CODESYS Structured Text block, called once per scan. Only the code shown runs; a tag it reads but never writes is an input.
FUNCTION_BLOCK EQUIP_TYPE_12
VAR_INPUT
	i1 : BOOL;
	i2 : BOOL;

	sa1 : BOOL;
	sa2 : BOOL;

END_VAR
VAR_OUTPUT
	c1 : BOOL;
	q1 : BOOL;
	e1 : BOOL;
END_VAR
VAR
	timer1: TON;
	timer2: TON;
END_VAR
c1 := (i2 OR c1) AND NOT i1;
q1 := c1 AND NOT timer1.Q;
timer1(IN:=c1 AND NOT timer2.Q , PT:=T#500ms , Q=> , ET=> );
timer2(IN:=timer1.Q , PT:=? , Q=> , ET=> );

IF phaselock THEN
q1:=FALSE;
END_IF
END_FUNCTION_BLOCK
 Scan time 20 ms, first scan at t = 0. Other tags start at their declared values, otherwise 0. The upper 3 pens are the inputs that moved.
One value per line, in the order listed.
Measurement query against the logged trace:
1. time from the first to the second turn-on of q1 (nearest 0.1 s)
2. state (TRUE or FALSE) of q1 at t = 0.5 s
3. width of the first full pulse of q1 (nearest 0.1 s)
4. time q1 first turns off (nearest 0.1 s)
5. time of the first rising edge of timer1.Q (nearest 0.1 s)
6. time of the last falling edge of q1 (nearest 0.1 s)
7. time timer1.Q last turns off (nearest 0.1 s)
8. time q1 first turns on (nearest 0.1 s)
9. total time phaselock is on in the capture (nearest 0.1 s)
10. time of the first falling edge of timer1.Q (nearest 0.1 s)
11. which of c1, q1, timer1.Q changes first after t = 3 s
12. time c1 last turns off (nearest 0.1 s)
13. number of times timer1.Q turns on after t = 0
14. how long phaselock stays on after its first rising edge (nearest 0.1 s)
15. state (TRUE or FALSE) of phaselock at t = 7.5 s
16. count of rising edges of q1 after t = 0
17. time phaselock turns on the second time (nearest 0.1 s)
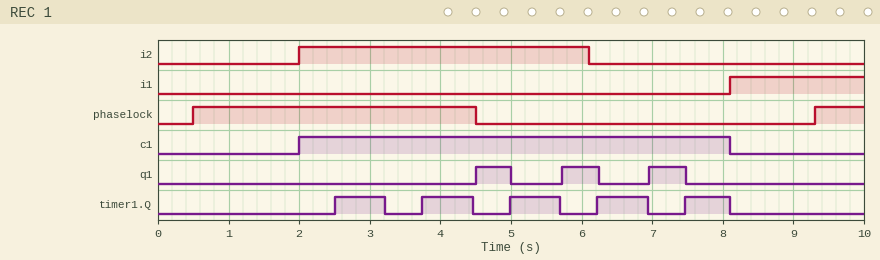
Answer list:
1.2 s
FALSE
0.5 s
5.0 s
2.5 s
7.5 s
8.1 s
4.5 s
4.7 s
3.2 s
timer1.Q
8.1 s
5
4.0 s
FALSE
3
9.3 s
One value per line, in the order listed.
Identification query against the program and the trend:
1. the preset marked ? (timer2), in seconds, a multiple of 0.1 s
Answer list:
0.7 s
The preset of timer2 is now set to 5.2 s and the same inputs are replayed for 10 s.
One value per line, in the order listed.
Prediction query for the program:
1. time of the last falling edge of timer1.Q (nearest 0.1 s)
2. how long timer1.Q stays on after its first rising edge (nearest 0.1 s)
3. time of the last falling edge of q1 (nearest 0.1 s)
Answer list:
7.7 s
5.2 s
8.1 s
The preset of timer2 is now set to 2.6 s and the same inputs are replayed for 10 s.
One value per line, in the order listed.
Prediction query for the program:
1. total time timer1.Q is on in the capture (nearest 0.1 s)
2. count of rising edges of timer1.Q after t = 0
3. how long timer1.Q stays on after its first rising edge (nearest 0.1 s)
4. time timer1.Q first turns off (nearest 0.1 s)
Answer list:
5.1 s
2
2.6 s
5.1 s
